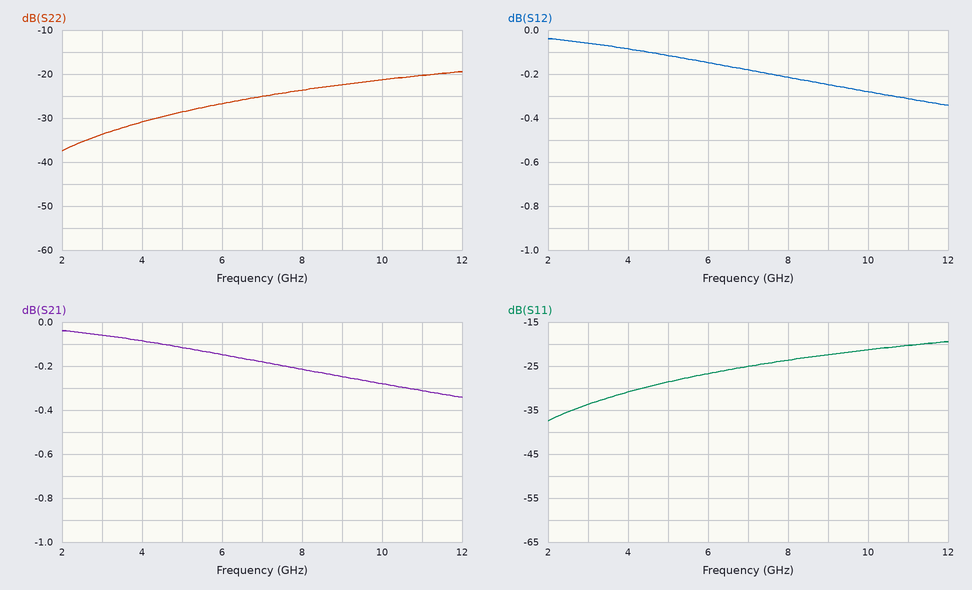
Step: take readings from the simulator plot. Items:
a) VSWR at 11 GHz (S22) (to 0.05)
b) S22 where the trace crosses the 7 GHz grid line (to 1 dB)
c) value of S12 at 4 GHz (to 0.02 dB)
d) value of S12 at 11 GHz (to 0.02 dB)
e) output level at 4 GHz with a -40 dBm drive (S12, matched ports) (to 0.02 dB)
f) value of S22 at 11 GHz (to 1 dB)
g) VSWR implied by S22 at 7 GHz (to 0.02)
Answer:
1.20
-25 dB
-0.08 dB
-0.32 dB
-40.08 dBm
-20 dB
1.12
